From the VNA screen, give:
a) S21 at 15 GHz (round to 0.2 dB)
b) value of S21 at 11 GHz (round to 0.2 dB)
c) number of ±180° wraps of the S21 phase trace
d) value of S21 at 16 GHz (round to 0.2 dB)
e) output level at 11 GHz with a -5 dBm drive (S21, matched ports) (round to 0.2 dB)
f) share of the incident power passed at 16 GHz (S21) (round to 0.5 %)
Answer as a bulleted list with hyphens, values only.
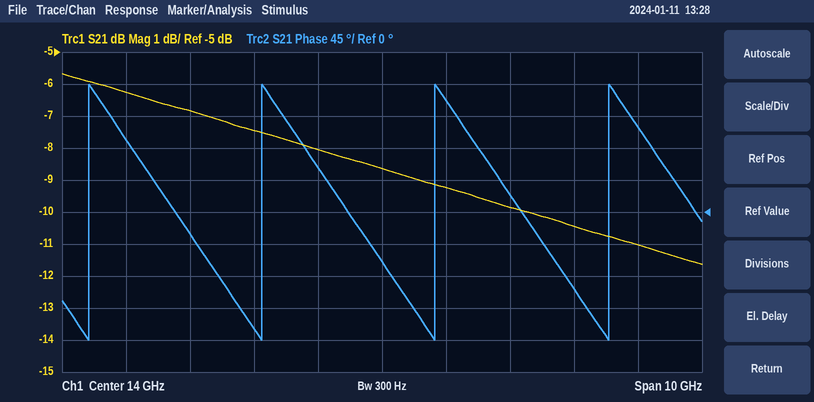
- -9.2 dB
- -6.8 dB
- 4
- -9.8 dB
- -11.8 dBm
- 10.5 %
